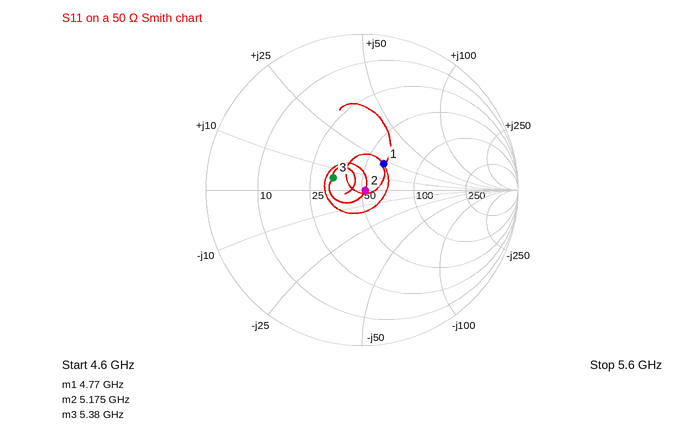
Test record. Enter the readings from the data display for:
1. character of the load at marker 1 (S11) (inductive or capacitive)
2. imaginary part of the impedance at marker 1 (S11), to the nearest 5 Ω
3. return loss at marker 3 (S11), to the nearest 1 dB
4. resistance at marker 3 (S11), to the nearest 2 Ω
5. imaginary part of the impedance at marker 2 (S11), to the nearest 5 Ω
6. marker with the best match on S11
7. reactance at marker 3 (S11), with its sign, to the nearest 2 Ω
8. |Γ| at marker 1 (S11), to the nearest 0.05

inductive
+20 Ω
14 dB
34 Ω
0 Ω
marker 2
+6 Ω
0.20
